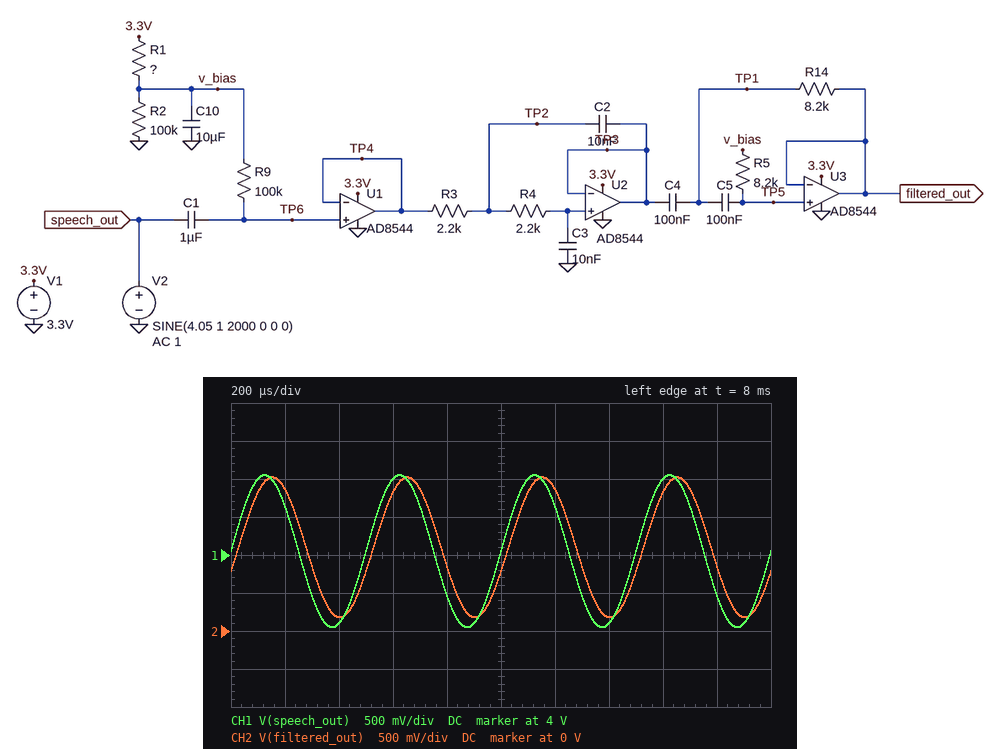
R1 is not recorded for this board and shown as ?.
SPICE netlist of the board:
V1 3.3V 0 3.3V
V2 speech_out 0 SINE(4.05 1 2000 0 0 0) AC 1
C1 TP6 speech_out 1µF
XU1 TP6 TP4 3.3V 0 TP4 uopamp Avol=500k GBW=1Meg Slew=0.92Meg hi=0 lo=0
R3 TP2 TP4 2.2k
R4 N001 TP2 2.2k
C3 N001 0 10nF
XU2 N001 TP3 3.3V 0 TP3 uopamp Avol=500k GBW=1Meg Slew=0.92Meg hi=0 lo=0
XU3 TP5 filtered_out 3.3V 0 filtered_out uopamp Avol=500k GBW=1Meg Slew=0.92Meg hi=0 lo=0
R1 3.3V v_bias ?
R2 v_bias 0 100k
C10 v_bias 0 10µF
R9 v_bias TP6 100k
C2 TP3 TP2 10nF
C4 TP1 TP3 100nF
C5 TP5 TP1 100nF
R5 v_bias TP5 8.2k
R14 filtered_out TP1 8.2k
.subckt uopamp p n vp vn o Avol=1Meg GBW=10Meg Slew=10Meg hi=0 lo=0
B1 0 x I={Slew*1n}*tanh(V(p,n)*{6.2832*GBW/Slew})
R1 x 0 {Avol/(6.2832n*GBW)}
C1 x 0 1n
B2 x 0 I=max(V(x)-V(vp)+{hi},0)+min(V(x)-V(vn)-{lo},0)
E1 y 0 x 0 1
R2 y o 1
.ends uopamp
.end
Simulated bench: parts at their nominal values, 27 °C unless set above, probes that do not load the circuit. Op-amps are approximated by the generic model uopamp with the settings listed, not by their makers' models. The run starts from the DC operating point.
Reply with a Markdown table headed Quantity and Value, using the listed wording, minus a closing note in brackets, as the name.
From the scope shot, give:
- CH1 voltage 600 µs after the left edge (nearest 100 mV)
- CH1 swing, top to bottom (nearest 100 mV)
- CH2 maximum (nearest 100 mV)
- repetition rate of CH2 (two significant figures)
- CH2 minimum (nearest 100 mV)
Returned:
| Quantity | Value |
|---|---|
| CH1 voltage 600 µs after the left edge | 5.0 V |
| CH1 swing, top to bottom | 2.0 V |
| CH2 maximum | 2.0 V |
| repetition rate of CH2 | 2.0 kHz |
| CH2 minimum | 200 mV |
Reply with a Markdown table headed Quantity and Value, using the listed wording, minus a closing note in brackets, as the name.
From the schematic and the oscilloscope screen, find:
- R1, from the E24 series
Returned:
| Quantity | Value |
|---|---|
| R1, from the E24 series | 200 kΩ |
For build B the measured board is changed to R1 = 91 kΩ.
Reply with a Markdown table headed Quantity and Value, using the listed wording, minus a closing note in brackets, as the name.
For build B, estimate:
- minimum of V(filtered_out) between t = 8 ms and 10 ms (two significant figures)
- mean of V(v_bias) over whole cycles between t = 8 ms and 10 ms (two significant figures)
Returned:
| Quantity | Value |
|---|---|
| minimum of V(filtered_out) between t = 8 ms and 10 ms | 810 mV |
| mean of V(v_bias) over whole cycles between t = 8 ms and 10 ms | 1.7 V |
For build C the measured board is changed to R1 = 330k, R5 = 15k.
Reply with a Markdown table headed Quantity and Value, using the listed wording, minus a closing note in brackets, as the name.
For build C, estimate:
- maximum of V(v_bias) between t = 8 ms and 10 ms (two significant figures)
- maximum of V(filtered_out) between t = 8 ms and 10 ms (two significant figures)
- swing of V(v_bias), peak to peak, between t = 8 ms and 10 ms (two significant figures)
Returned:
| Quantity | Value |
|---|---|
| maximum of V(v_bias) between t = 8 ms and 10 ms | 770 mV |
| maximum of V(filtered_out) between t = 8 ms and 10 ms | 1.7 V |
| swing of V(v_bias), peak to peak, between t = 8 ms and 10 ms | 1.1 mV |
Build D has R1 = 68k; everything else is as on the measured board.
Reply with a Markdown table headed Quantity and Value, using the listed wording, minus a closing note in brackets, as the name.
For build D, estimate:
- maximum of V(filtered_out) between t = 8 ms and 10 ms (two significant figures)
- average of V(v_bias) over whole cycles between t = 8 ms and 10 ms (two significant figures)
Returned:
| Quantity | Value |
|---|---|
| maximum of V(filtered_out) between t = 8 ms and 10 ms | 2.9 V |
| average of V(v_bias) over whole cycles between t = 8 ms and 10 ms | 2.0 V |
